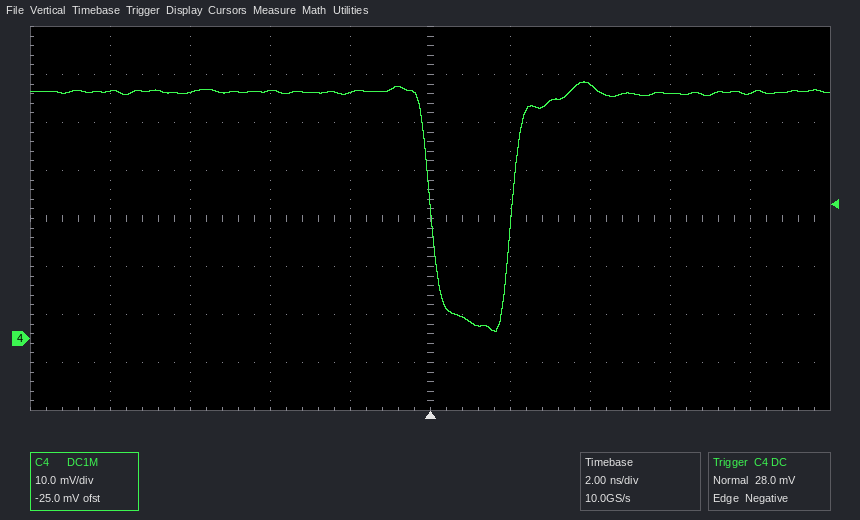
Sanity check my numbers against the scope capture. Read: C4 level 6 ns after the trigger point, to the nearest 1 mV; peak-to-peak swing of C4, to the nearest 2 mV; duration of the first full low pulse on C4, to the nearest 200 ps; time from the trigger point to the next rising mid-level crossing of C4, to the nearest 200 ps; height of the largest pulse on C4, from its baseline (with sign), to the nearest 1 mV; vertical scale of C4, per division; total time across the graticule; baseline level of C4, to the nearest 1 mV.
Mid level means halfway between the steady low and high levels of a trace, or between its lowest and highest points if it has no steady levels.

51 mV
52 mV
2.0 ns
2.0 ns
-50 mV
10 mV
20 ns
51 mV
